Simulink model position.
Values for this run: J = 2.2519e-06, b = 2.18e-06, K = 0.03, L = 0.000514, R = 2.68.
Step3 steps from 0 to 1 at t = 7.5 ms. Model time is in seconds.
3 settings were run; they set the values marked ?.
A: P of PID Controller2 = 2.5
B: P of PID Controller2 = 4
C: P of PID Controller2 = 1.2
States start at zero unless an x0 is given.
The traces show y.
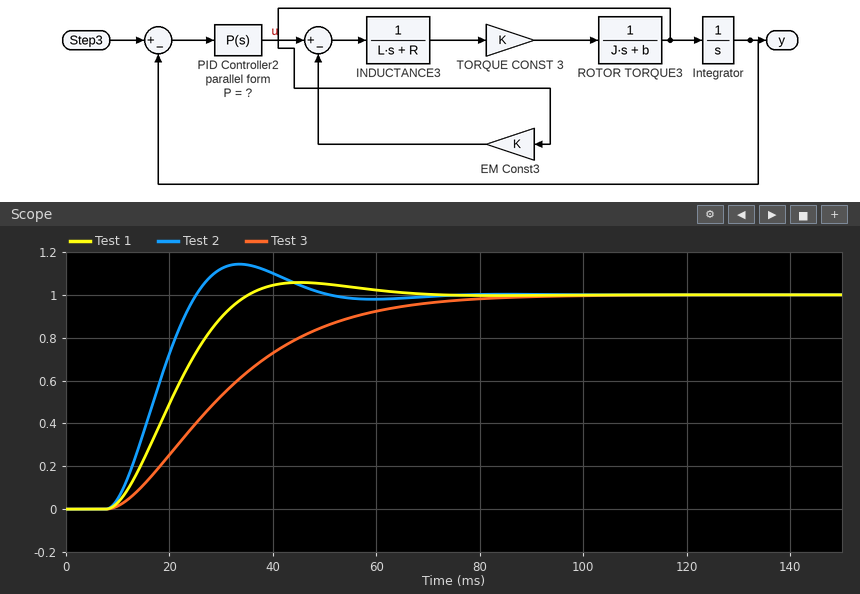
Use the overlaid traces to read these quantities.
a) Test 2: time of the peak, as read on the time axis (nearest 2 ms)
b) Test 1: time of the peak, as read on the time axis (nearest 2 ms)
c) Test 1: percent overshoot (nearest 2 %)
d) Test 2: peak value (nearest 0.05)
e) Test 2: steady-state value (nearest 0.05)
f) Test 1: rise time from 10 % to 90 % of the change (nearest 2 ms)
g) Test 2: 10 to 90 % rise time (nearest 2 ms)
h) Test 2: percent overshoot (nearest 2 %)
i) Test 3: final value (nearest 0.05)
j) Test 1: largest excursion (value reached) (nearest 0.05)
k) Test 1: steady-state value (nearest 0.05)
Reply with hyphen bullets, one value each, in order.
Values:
- 34 ms
- 46 ms
- 6 %
- 1.15
- 1.00
- 18 ms
- 12 ms
- 14 %
- 1.00
- 1.05
- 1.00
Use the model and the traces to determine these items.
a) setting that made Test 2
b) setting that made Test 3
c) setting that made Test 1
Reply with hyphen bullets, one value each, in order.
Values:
- B
- C
- A
